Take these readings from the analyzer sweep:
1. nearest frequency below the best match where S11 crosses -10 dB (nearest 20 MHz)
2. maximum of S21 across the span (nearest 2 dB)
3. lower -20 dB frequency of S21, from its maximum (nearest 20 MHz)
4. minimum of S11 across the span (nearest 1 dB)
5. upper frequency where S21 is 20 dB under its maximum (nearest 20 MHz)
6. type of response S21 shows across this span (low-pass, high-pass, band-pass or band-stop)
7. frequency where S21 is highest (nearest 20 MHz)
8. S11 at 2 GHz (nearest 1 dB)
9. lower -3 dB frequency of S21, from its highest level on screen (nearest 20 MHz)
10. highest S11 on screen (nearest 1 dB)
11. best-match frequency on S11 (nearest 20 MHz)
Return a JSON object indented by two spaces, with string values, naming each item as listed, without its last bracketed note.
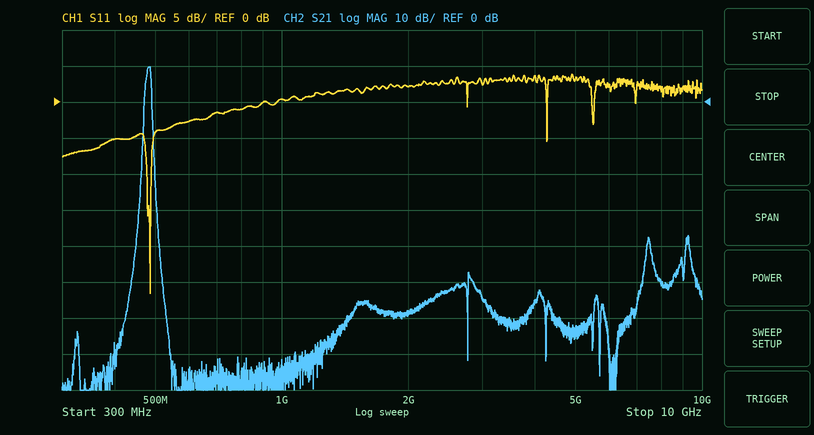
{
  "nearest frequency below the best match where S11 crosses -10 dB": "480 MHz",
  "maximum of S21 across the span": "10 dB",
  "lower -20 dB frequency of S21, from its maximum": "460 MHz",
  "minimum of S11 across the span": "-27 dB",
  "upper frequency where S21 is 20 dB under its maximum": "500 MHz",
  "type of response S21 shows across this span": "band-pass",
  "frequency where S21 is highest": "480 MHz",
  "S11 at 2 GHz": "2 dB",
  "lower -3 dB frequency of S21, from its highest level on screen": "480 MHz",
  "highest S11 on screen": "4 dB",
  "best-match frequency on S11": "480 MHz"
}
